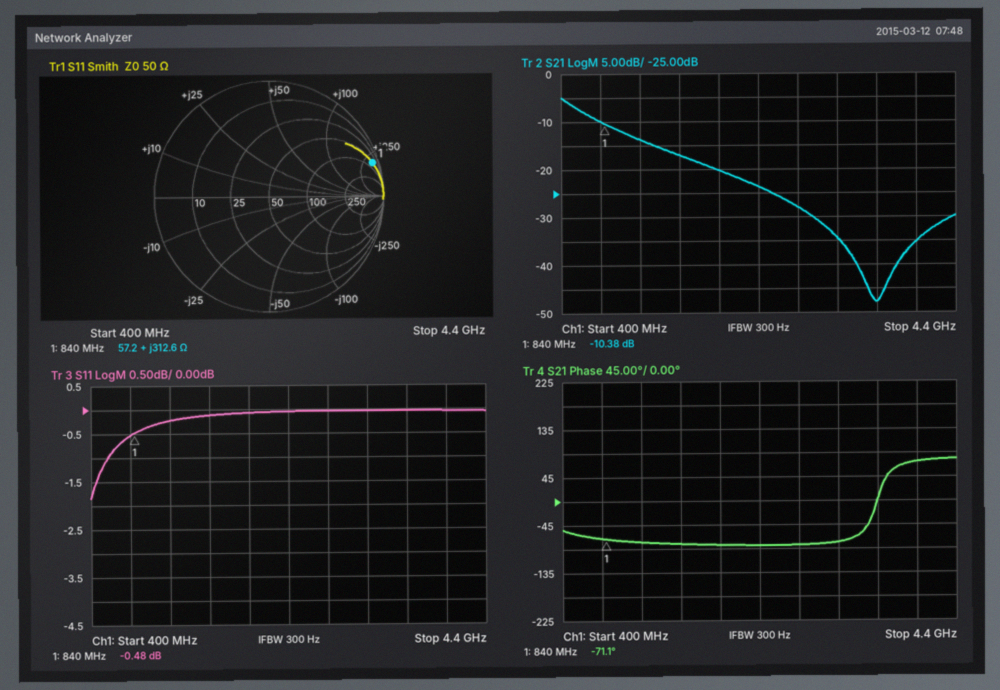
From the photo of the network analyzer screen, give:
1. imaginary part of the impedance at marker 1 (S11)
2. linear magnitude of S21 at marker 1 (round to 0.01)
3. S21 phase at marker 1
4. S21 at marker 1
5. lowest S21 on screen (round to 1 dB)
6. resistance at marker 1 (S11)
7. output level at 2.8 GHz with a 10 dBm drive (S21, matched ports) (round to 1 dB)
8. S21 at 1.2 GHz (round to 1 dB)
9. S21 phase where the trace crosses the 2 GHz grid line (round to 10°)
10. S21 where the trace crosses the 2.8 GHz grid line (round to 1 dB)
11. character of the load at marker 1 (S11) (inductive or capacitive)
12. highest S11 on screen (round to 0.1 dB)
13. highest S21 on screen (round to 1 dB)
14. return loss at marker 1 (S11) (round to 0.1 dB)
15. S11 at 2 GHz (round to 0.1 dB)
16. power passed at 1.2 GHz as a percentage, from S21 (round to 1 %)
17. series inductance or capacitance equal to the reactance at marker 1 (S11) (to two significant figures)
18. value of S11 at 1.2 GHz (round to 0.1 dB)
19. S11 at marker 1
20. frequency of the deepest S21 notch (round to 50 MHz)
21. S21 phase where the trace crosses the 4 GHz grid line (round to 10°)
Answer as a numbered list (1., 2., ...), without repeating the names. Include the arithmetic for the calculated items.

1. +312.6 Ω
2. 10^(-10.38/20) ≈ 0.30
3. -71.1°
4. -10.38 dB
5. -48 dB
6. 57.2 Ω
7. 10 dBm + (-28 dB) = -18 dBm
8. -14 dB
9. -80°
10. -28 dB
11. inductive
12. 0.0 dB
13. -5 dB
14. 0.5 dB
15. -0.1 dB
16. 10^(-14/10) ≈ 4 %
17. L = 312.6 Ω/(2π × 840 MHz) ≈ 59 nH
18. -0.2 dB
19. -0.48 dB
20. 3.60 GHz
21. 70°
